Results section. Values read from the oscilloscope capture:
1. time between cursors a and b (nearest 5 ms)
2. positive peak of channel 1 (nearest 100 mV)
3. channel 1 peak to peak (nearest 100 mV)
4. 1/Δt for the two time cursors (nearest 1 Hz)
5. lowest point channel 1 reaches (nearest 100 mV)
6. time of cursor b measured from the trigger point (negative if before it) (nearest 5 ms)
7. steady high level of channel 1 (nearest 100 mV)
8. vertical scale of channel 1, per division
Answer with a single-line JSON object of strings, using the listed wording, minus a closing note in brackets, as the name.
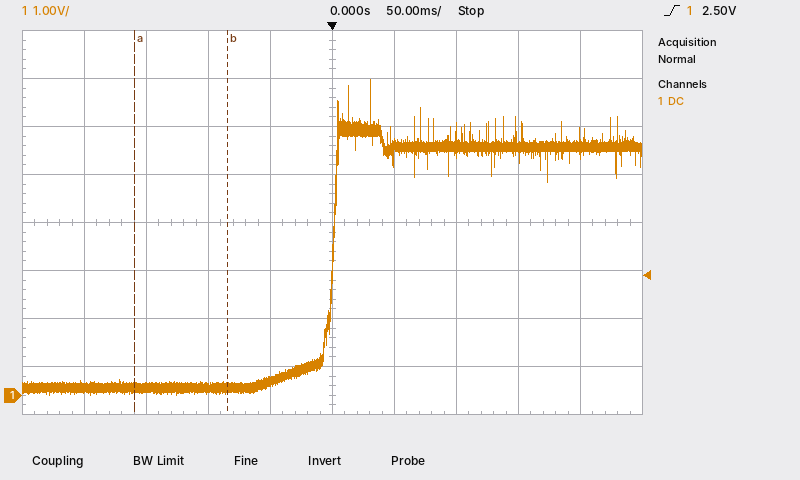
{"time between cursors a and b": "75 ms", "positive peak of channel 1": "6.6 V", "channel 1 peak to peak": "6.6 V", "1/Δt for the two time cursors": "13 Hz", "lowest point channel 1 reaches": "0.0 V", "time of cursor b measured from the trigger point (negative if before it)": "-85 ms", "steady high level of channel 1": "5.2 V", "vertical scale of channel 1, per division": "1 V"}
